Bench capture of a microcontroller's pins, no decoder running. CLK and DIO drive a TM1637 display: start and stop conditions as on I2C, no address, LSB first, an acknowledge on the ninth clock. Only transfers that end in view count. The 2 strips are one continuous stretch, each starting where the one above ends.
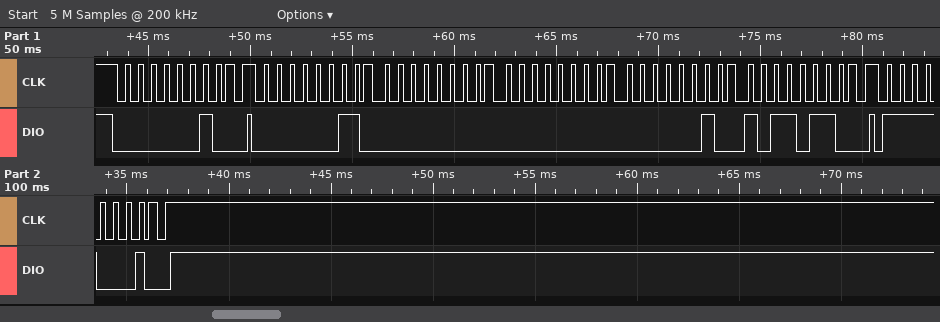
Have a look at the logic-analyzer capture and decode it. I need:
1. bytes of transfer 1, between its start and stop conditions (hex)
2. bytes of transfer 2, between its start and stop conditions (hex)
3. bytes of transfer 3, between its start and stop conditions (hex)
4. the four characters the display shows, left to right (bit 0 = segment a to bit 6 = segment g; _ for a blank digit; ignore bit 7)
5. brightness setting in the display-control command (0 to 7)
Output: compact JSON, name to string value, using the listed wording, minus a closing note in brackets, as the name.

{"bytes of transfer 1, between its start and stop conditions": "40", "bytes of transfer 2, between its start and stop conditions": "C0 00 00 40 6D", "bytes of transfer 3, between its start and stop conditions": "8F", "the four characters the display shows, left to right": "__-5", "brightness setting in the display-control command": "7"}
